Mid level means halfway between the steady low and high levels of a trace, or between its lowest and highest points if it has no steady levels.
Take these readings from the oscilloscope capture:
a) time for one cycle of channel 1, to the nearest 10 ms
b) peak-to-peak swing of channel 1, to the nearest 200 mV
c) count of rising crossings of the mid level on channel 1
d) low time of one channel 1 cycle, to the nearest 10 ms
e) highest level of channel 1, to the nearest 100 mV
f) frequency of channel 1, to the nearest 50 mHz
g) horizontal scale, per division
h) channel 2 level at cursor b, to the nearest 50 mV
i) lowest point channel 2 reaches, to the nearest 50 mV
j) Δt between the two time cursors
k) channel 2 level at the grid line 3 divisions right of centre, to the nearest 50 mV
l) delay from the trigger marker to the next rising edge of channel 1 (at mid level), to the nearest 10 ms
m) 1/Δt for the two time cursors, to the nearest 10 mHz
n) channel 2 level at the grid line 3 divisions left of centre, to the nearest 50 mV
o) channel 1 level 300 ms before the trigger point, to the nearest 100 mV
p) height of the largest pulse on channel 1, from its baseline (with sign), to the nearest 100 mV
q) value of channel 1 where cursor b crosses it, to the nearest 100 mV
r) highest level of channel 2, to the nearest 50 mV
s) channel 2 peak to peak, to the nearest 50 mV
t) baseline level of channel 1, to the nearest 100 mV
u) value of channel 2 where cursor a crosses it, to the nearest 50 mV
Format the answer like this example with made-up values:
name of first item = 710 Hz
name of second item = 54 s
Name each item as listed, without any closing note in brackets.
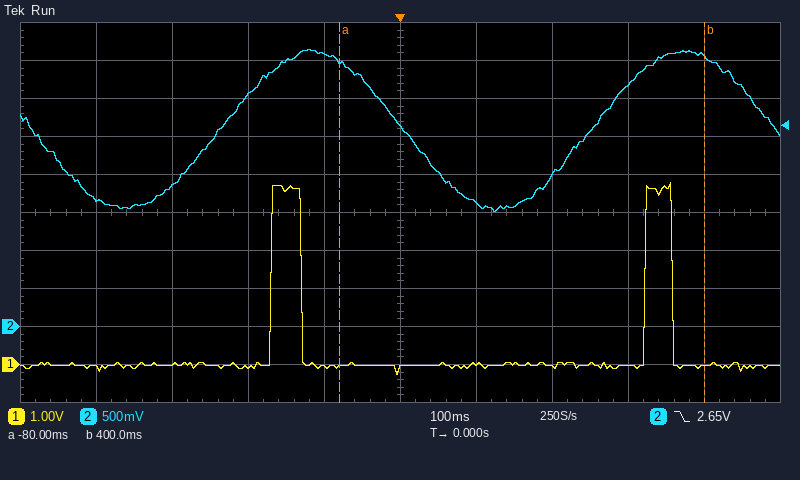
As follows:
time for one cycle of channel 1, to the nearest 10 ms = 490 ms
peak-to-peak swing of channel 1, to the nearest 200 mV = 5.0 V
count of rising crossings of the mid level on channel 1 = 2
low time of one channel 1 cycle, to the nearest 10 ms = 450 ms
highest level of channel 1, to the nearest 100 mV = 4.8 V
frequency of channel 1, to the nearest 50 mHz = 2.05 Hz
horizontal scale, per division = 100 ms
channel 2 level at cursor b, to the nearest 50 mV = 3.55 V
lowest point channel 2 reaches, to the nearest 50 mV = 1.50 V
Δt between the two time cursors = 480 ms
channel 2 level at the grid line 3 divisions right of centre, to the nearest 50 mV = 3.20 V
delay from the trigger marker to the next rising edge of channel 1 (at mid level), to the nearest 10 ms = 320 ms
1/Δt for the two time cursors, to the nearest 10 mHz = 2.08 Hz
channel 2 level at the grid line 3 divisions left of centre, to the nearest 50 mV = 1.85 V
channel 1 level 300 ms before the trigger point, to the nearest 100 mV = 0.0 V
height of the largest pulse on channel 1, from its baseline (with sign), to the nearest 100 mV = +4.8 V
value of channel 1 where cursor b crosses it, to the nearest 100 mV = 0.0 V
highest level of channel 2, to the nearest 50 mV = 3.65 V
channel 2 peak to peak, to the nearest 50 mV = 2.15 V
baseline level of channel 1, to the nearest 100 mV = 0.0 V
value of channel 2 where cursor a crosses it, to the nearest 50 mV = 3.50 V
